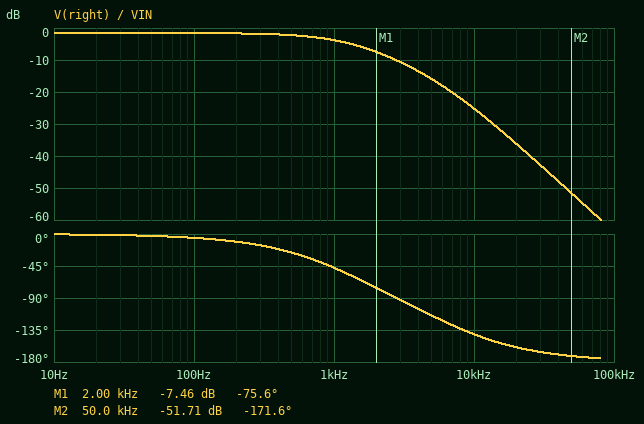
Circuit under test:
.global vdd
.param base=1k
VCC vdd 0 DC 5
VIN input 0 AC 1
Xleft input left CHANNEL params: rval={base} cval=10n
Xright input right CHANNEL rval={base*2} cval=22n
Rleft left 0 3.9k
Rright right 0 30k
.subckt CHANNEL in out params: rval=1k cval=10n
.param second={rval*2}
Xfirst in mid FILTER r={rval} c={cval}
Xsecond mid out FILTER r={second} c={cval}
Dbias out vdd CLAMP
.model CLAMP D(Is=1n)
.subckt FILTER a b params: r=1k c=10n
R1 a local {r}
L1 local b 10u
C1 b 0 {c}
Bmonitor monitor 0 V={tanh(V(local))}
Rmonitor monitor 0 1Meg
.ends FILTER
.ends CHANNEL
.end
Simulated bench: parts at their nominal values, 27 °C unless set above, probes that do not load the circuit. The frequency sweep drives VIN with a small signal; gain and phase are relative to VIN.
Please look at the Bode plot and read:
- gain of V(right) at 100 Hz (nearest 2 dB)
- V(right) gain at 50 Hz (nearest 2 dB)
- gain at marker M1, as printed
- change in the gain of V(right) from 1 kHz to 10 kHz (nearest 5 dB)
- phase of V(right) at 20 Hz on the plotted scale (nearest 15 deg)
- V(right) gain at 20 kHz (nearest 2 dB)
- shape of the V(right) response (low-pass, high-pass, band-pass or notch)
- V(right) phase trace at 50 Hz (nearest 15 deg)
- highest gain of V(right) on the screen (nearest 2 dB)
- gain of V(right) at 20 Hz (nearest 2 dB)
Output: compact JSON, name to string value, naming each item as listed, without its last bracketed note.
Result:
{"gain of V(right) at 100 Hz": "-2 dB", "V(right) gain at 50 Hz": "-2 dB", "gain at marker M1, as printed": "-7.46 dB", "change in the gain of V(right) from 1 kHz to 10 kHz": "-20 dB", "phase of V(right) at 20 Hz on the plotted scale": "0 deg", "V(right) gain at 20 kHz": "-36 dB", "shape of the V(right) response": "low-pass", "V(right) phase trace at 50 Hz": "0 deg", "highest gain of V(right) on the screen": "-2 dB", "gain of V(right) at 20 Hz": "-2 dB"}
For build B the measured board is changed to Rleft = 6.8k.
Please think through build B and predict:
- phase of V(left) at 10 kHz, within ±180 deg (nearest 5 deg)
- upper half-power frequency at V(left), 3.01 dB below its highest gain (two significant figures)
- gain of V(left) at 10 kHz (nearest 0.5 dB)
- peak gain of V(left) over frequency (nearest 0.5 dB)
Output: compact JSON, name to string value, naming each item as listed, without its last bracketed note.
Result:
{"phase of V(left) at 10 kHz, within ±180 deg": "-75 deg", "upper half-power frequency at V(left), 3.01 dB below its highest gain": "6.3 kHz", "gain of V(left) at 10 kHz": "-9.0 dB", "peak gain of V(left) over frequency": "-3.0 dB"}
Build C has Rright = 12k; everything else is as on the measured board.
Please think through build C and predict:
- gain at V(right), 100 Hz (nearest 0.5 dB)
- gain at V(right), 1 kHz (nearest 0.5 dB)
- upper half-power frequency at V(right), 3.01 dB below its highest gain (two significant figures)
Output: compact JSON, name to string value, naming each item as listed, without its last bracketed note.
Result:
{"gain at V(right), 100 Hz": "-3.5 dB", "gain at V(right), 1 kHz": "-5.0 dB", "upper half-power frequency at V(right), 3.01 dB below its highest gain": "1.5 kHz"}
